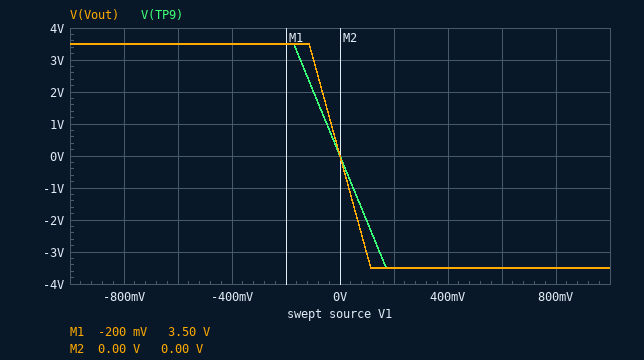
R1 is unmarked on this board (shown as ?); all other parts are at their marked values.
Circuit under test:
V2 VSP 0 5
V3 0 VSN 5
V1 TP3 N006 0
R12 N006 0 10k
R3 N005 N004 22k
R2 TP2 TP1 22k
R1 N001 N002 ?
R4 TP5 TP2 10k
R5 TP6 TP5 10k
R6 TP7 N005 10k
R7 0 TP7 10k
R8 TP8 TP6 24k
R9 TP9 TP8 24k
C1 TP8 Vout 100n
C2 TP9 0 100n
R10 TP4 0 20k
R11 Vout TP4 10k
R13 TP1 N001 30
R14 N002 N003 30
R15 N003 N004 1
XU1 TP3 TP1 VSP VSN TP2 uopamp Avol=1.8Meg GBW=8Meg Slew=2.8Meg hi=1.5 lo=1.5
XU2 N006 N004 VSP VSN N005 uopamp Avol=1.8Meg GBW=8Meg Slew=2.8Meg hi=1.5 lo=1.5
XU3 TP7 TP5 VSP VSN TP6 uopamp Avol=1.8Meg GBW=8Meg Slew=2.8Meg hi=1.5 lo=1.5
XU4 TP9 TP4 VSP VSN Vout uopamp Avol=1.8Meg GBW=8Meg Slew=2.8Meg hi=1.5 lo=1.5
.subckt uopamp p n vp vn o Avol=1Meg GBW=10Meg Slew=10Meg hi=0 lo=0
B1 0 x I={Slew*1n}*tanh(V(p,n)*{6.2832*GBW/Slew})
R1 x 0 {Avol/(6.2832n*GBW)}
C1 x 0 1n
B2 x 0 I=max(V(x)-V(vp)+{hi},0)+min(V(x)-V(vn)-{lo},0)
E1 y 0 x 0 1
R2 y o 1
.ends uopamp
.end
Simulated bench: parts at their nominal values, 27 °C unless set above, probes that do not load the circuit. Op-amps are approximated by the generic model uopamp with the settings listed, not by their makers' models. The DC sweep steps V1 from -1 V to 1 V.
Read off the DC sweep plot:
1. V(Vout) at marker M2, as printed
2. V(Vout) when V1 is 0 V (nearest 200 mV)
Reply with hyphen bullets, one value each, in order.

- 0.00 V
- 0 V
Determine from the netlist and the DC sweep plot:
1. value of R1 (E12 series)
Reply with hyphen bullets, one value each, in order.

- 2.2 kΩ
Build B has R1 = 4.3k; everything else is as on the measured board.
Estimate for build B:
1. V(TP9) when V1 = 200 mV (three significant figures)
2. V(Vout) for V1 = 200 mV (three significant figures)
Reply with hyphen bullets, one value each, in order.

- -2.22 V
- -3.33 V
